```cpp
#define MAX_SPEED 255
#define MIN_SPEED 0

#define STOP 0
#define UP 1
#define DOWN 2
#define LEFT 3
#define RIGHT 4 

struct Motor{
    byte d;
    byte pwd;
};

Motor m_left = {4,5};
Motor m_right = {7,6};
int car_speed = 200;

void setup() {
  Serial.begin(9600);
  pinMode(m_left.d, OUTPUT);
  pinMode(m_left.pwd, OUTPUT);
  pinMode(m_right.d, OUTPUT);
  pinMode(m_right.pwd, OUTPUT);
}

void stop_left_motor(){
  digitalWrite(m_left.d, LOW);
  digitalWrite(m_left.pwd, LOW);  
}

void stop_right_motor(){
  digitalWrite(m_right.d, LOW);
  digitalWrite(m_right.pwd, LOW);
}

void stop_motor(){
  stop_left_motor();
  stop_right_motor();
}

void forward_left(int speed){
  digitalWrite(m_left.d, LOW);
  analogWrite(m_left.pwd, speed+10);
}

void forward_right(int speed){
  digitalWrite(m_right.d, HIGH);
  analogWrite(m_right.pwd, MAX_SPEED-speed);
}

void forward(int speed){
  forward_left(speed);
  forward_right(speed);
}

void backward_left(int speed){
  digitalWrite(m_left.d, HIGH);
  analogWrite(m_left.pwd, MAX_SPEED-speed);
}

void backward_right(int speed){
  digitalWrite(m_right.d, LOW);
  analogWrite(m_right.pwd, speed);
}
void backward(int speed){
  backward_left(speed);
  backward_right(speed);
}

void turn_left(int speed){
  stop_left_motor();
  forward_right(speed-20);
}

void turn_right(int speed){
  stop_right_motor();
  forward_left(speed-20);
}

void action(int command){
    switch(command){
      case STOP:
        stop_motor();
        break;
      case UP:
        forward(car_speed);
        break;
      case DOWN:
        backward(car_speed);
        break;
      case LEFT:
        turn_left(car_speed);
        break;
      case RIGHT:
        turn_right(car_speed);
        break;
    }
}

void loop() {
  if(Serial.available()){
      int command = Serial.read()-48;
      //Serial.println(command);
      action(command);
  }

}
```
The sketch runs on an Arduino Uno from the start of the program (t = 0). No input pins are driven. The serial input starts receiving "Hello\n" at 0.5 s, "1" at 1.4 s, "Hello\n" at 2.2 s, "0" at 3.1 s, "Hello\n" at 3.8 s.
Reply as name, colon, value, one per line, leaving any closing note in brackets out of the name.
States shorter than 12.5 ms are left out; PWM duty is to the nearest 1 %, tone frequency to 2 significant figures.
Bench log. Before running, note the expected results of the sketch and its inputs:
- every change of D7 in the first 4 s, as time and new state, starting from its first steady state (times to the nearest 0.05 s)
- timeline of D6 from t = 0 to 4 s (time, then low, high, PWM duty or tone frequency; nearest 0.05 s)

every change of D7 in the first 4 s, as time and new state, starting from its first steady state: 0 s low; 1.4 s high; 3.1 s low
timeline of D6 from t = 0 to 4 s: 0 s low; 1.4 s PWM 22 %; 3.1 s low
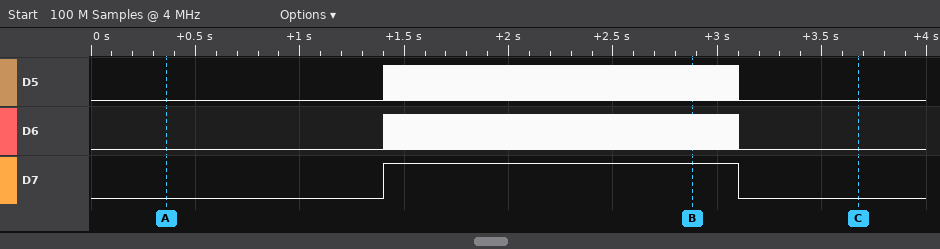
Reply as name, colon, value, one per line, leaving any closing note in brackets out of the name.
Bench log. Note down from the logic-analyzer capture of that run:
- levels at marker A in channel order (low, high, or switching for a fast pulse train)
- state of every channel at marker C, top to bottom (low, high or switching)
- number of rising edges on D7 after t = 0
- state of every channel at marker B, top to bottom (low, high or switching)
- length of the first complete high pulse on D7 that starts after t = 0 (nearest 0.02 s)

levels at marker A in channel order: D5 low, D6 low, D7 low
state of every channel at marker C, top to bottom: D5 low, D6 low, D7 low
number of rising edges on D7 after t = 0: 1
state of every channel at marker B, top to bottom: D5 switching, D6 switching, D7 high
length of the first complete high pulse on D7 that starts after t = 0: 1.70 s
